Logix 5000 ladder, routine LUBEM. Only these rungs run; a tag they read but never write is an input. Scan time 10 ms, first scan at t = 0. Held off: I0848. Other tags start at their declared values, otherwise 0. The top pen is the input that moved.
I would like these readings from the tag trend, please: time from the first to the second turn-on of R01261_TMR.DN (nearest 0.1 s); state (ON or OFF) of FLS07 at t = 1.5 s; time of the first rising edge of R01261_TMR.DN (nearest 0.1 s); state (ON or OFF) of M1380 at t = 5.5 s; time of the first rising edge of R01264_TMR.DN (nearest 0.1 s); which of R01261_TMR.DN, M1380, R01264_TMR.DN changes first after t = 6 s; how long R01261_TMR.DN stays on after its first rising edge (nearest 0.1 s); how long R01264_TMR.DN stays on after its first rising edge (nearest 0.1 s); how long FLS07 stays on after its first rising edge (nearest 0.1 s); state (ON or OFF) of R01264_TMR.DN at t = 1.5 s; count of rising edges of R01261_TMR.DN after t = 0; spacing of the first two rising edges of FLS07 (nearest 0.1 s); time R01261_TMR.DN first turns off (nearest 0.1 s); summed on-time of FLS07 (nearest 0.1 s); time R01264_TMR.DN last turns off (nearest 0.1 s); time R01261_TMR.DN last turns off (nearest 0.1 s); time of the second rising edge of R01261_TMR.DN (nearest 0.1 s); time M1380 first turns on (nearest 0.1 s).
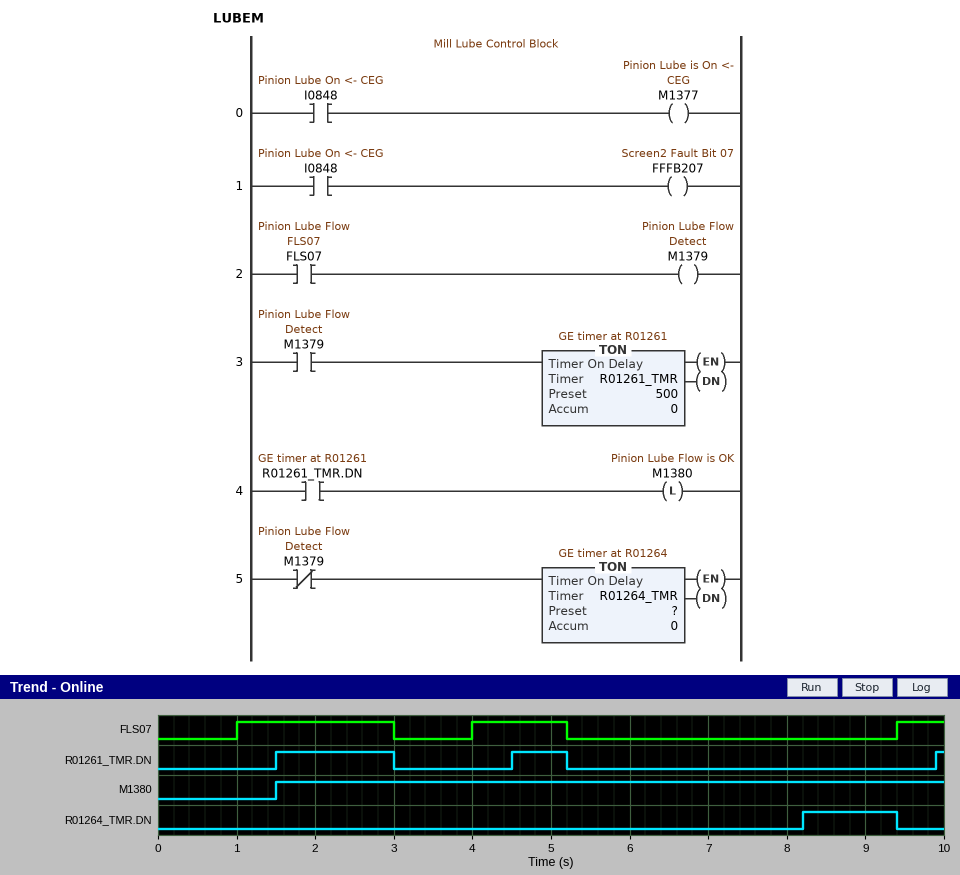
3.0 s
ON
1.5 s
ON
8.2 s
R01264_TMR.DN
1.5 s
1.2 s
2.0 s
OFF
3
3.0 s
3.0 s
3.8 s
9.4 s
5.2 s
4.5 s
1.5 s
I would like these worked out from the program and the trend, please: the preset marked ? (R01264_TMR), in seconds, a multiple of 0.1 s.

3.0 s
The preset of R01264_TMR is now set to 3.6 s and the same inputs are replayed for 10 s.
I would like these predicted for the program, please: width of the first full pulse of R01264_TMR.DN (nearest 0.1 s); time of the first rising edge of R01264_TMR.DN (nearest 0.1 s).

0.6 s
8.8 s
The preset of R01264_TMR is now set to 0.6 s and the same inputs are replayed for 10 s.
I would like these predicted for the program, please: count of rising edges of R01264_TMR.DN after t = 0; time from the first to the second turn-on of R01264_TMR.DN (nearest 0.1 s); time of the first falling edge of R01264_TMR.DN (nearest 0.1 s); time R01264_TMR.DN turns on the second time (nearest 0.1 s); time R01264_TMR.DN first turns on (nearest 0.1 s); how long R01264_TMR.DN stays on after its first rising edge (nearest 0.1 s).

3
3.0 s
1.0 s
3.6 s
0.6 s
0.4 s
